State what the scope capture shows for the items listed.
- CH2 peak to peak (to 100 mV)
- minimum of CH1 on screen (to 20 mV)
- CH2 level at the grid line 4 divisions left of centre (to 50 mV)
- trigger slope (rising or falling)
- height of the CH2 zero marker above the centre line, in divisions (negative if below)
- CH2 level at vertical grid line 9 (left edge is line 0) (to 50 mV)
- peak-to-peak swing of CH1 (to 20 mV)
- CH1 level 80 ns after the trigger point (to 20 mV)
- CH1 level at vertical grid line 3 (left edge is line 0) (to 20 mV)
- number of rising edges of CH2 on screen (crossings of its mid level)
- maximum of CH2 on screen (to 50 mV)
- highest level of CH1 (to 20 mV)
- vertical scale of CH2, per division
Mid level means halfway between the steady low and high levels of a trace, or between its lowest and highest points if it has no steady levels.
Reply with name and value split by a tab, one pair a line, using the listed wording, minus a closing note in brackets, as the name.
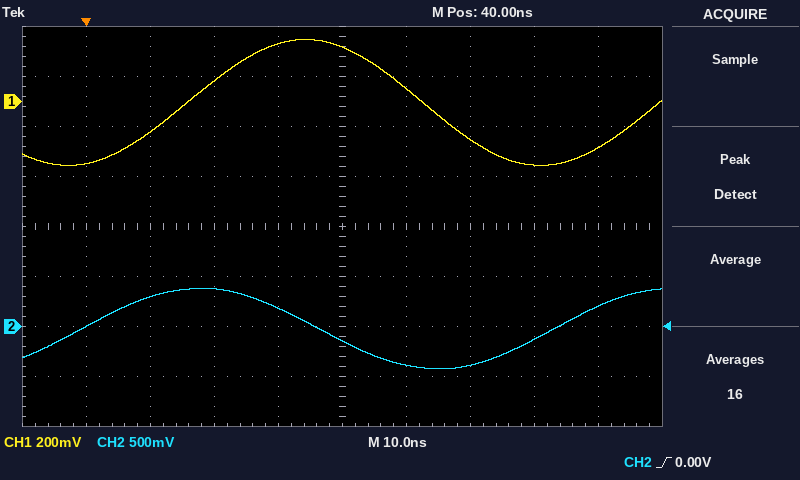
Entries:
CH2 peak to peak	800 mV
minimum of CH1 on screen	-260 mV
CH2 level at the grid line 4 divisions left of centre	0 mV
trigger slope	rising
height of the CH2 zero marker above the centre line, in divisions	-2.0 div
CH2 level at vertical grid line 9 (left edge is line 0)	200 mV
peak-to-peak swing of CH1	500 mV
CH1 level 80 ns after the trigger point	-180 mV
CH1 level at vertical grid line 3 (left edge is line 0)	80 mV
number of rising edges of CH2 on screen	2
maximum of CH2 on screen	400 mV
highest level of CH1	240 mV
vertical scale of CH2, per division	500 mV
